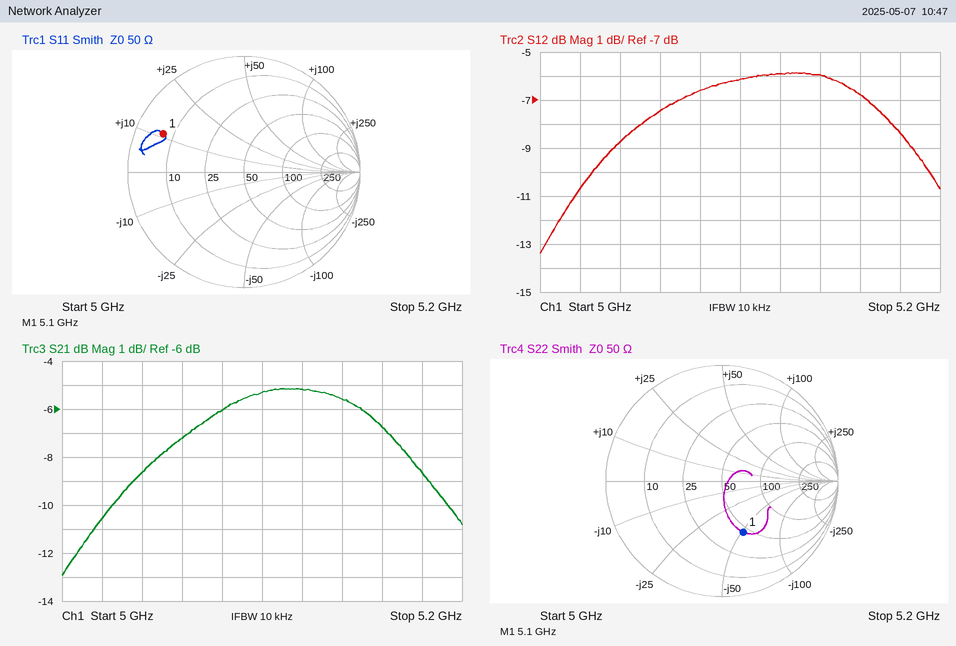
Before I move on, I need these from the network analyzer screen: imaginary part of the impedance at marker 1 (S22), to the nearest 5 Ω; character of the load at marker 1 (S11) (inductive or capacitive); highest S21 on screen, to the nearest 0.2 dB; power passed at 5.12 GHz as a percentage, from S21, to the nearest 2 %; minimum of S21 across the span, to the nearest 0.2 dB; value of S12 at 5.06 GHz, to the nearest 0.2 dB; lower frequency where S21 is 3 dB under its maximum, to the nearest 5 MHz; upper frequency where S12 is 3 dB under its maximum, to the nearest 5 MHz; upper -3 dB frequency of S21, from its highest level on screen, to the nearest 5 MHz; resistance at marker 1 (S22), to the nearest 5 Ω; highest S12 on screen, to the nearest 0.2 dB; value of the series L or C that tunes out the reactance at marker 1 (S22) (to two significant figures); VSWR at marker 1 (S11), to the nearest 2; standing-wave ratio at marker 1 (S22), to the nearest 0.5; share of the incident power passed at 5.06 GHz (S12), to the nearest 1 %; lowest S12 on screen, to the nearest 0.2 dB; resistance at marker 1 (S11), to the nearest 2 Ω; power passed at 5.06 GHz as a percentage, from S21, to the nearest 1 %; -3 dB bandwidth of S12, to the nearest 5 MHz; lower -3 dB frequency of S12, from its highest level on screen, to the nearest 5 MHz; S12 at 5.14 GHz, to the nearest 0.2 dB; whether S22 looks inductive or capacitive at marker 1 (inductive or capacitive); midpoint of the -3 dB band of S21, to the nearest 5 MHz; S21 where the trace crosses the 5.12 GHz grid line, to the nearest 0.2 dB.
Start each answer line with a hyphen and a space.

- -50 Ω
- inductive
- -5.2 dB
- 30 %
- -13.0 dB
- -7.4 dB
- 5.045 GHz
- 5.185 GHz
- 5.175 GHz
- 45 Ω
- -5.8 dB
- 1.6 nH
- 8
- 3.0
- 18 %
- -13.4 dB
- 6 Ω
- 19 %
- 145 MHz
- 5.040 GHz
- -6.0 dB
- capacitive
- 5.110 GHz
- -5.2 dB
